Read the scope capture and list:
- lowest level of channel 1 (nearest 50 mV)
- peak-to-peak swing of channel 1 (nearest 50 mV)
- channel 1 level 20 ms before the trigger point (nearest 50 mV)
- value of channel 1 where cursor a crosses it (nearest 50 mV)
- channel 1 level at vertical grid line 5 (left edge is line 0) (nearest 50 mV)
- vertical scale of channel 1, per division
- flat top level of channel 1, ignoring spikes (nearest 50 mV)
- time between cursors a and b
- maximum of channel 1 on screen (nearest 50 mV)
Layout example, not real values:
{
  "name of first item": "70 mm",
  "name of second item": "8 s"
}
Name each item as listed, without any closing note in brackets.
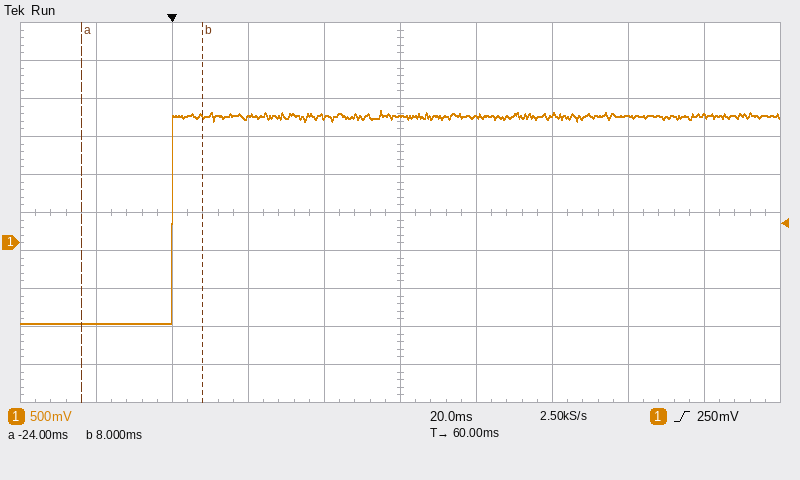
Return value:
{
  "lowest level of channel 1": "-1.05 V",
  "peak-to-peak swing of channel 1": "2.80 V",
  "channel 1 level 20 ms before the trigger point": "-1.05 V",
  "value of channel 1 where cursor a crosses it": "-1.05 V",
  "channel 1 level at vertical grid line 5 (left edge is line 0)": "1.65 V",
  "vertical scale of channel 1, per division": "500 mV",
  "flat top level of channel 1, ignoring spikes": "1.65 V",
  "time between cursors a and b": "32 ms",
  "maximum of channel 1 on screen": "1.75 V"
}
